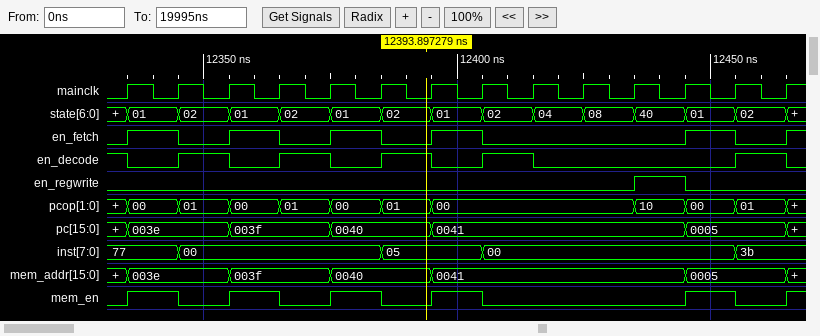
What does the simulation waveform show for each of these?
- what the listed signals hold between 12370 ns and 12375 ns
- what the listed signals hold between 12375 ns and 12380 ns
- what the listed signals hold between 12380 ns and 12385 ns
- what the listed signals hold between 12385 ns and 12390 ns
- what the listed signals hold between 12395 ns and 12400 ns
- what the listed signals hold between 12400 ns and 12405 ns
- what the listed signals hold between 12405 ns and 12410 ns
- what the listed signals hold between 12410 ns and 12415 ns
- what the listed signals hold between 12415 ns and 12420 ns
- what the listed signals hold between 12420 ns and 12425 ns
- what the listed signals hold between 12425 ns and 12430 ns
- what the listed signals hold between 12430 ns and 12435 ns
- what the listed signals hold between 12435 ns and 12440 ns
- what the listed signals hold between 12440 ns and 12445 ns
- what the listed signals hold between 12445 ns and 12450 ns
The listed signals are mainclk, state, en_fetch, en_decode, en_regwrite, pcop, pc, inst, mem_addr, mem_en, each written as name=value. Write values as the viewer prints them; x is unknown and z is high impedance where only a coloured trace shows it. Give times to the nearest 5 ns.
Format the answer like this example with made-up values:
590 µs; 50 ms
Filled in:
mainclk=0, state=02, en_fetch=0, en_decode=1, en_regwrite=0, pcop=01, pc=003f, inst=00, mem_addr=003f, mem_en=0; mainclk=1, state=01, en_fetch=1, en_decode=0, en_regwrite=0, pcop=00, pc=0040, inst=00, mem_addr=0040, mem_en=1; mainclk=0, state=01, en_fetch=1, en_decode=0, en_regwrite=0, pcop=00, pc=0040, inst=00, mem_addr=0040, mem_en=1; mainclk=1, state=02, en_fetch=0, en_decode=1, en_regwrite=0, pcop=01, pc=0040, inst=05, mem_addr=0040, mem_en=0; mainclk=1, state=01, en_fetch=1, en_decode=0, en_regwrite=0, pcop=00, pc=0041, inst=05, mem_addr=0041, mem_en=1; mainclk=0, state=01, en_fetch=1, en_decode=0, en_regwrite=0, pcop=00, pc=0041, inst=05, mem_addr=0041, mem_en=1; mainclk=1, state=02, en_fetch=0, en_decode=1, en_regwrite=0, pcop=00, pc=0041, inst=00, mem_addr=0041, mem_en=0; mainclk=0, state=02, en_fetch=0, en_decode=1, en_regwrite=0, pcop=00, pc=0041, inst=00, mem_addr=0041, mem_en=0; mainclk=1, state=04, en_fetch=0, en_decode=0, en_regwrite=0, pcop=00, pc=0041, inst=00, mem_addr=0041, mem_en=0; mainclk=0, state=04, en_fetch=0, en_decode=0, en_regwrite=0, pcop=00, pc=0041, inst=00, mem_addr=0041, mem_en=0; mainclk=1, state=08, en_fetch=0, en_decode=0, en_regwrite=0, pcop=00, pc=0041, inst=00, mem_addr=0041, mem_en=0; mainclk=0, state=08, en_fetch=0, en_decode=0, en_regwrite=0, pcop=00, pc=0041, inst=00, mem_addr=0041, mem_en=0; mainclk=1, state=40, en_fetch=0, en_decode=0, en_regwrite=1, pcop=10, pc=0041, inst=00, mem_addr=0041, mem_en=0; mainclk=0, state=40, en_fetch=0, en_decode=0, en_regwrite=1, pcop=10, pc=0041, inst=00, mem_addr=0041, mem_en=0; mainclk=1, state=01, en_fetch=1, en_decode=0, en_regwrite=0, pcop=00, pc=0005, inst=00, mem_addr=0005, mem_en=1
